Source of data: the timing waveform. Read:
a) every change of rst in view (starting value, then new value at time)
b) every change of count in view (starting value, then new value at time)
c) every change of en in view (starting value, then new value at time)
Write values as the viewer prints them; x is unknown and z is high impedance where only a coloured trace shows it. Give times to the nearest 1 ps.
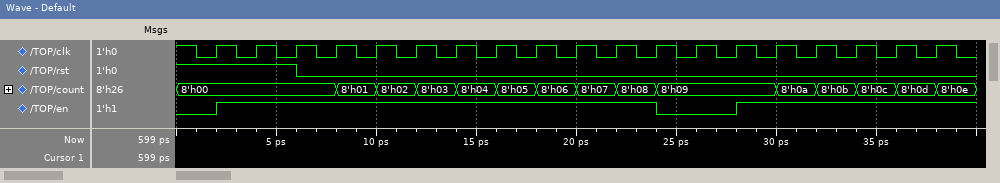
1, 0 at 6 ps
8'h00, 8'h01 at 8 ps, 8'h02 at 10 ps, 8'h03 at 12 ps, 8'h04 at 14 ps, 8'h05 at 16 ps, 8'h06 at 18 ps, 8'h07 at 20 ps, 8'h08 at 22 ps, 8'h09 at 24 ps, 8'h0a at 30 ps, 8'h0b at 32 ps, 8'h0c at 34 ps, 8'h0d at 36 ps, 8'h0e at 38 ps
0, 1 at 2 ps, 0 at 24 ps, 1 at 28 ps
